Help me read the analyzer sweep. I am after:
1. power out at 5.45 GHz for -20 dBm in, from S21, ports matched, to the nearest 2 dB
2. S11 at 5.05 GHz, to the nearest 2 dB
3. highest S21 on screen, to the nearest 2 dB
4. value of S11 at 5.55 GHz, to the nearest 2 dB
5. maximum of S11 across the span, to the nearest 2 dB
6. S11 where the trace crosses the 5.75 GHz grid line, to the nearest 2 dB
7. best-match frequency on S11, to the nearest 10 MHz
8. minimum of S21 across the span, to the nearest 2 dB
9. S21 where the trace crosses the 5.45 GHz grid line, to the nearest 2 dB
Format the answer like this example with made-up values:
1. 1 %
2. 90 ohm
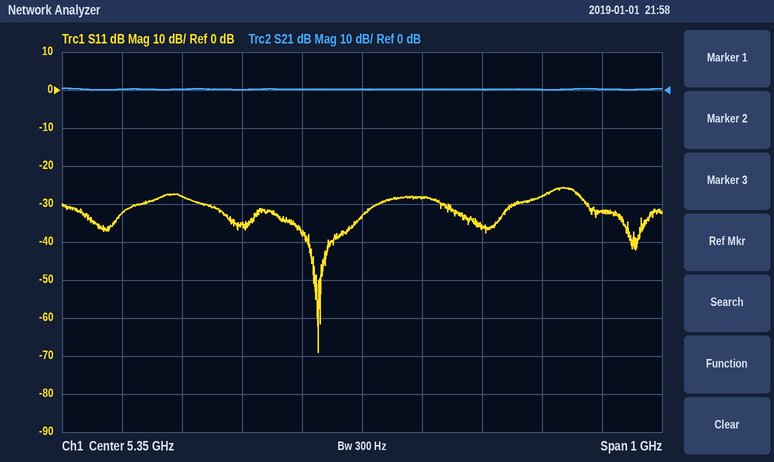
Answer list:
1. -20 dBm
2. -28 dB
3. 0 dB
4. -36 dB
5. -26 dB
6. -32 dB
7. 5.28 GHz
8. 0 dB
9. 0 dB
